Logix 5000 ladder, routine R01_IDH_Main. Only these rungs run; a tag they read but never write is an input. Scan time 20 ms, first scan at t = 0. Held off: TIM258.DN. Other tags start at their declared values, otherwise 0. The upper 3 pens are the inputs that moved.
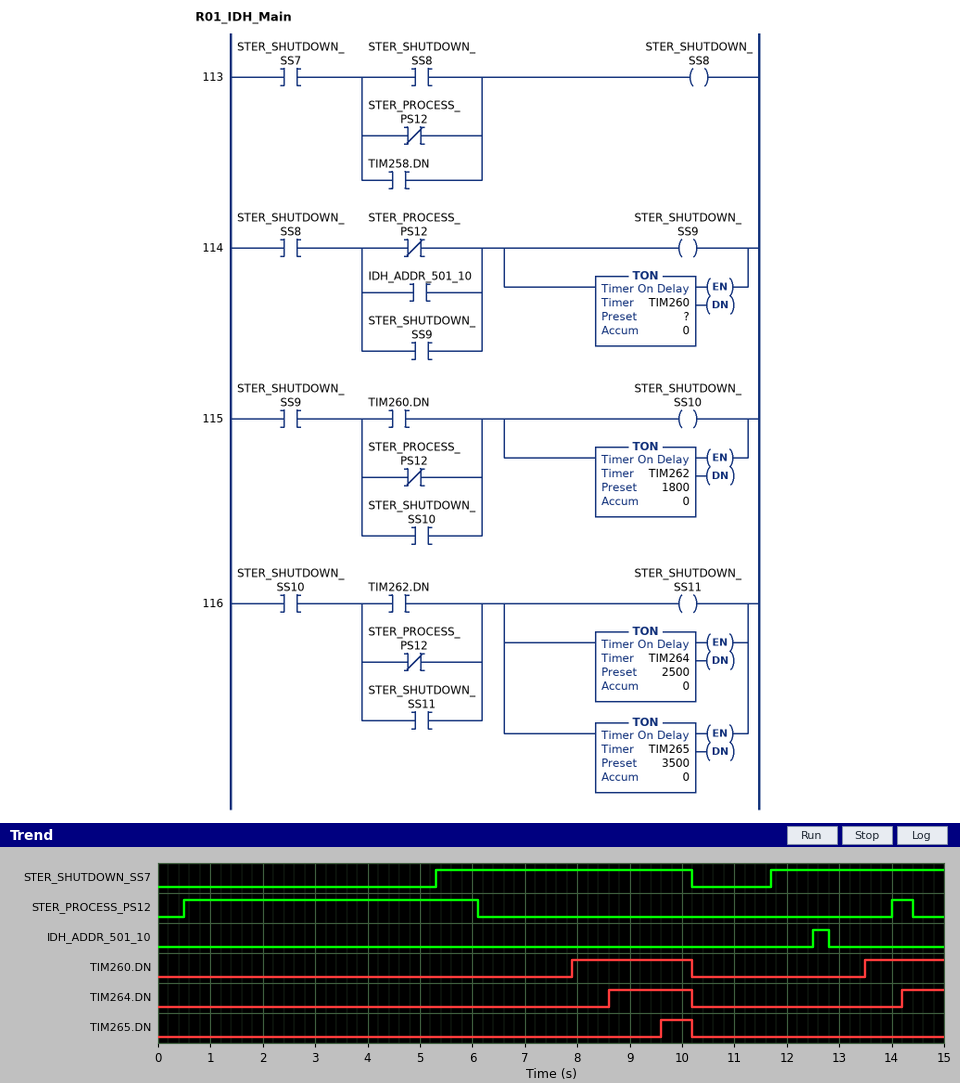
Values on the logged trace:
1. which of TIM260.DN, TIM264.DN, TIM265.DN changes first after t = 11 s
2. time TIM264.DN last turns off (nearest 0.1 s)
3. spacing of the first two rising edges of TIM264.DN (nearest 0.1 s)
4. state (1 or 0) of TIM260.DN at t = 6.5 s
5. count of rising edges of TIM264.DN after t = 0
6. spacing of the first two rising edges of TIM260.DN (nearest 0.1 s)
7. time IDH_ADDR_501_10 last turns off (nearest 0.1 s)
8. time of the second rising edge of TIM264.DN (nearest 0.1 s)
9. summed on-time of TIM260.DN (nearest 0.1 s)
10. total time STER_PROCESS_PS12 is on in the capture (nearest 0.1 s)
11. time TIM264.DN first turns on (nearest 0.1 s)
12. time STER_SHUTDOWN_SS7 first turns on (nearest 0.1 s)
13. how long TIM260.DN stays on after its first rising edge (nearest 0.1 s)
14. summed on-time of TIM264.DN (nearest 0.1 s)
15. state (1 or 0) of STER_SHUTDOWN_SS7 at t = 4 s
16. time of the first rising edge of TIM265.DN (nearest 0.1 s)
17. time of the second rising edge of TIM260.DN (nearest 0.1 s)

TIM260.DN
10.2 s
5.6 s
0
2
5.6 s
12.8 s
14.2 s
3.8 s
6.0 s
8.6 s
5.3 s
2.3 s
2.4 s
0
9.6 s
13.5 s
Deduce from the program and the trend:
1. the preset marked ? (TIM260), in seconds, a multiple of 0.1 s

1.8 s
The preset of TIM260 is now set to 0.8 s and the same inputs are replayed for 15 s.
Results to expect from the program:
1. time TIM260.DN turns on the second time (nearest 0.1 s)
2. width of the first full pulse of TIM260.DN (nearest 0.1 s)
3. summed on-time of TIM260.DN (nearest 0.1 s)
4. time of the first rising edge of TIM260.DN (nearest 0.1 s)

12.5 s
3.3 s
5.8 s
6.9 s
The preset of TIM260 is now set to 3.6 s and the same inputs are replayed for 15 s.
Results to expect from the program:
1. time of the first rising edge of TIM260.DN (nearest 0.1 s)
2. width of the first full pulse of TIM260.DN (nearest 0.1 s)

9.7 s
0.5 s
